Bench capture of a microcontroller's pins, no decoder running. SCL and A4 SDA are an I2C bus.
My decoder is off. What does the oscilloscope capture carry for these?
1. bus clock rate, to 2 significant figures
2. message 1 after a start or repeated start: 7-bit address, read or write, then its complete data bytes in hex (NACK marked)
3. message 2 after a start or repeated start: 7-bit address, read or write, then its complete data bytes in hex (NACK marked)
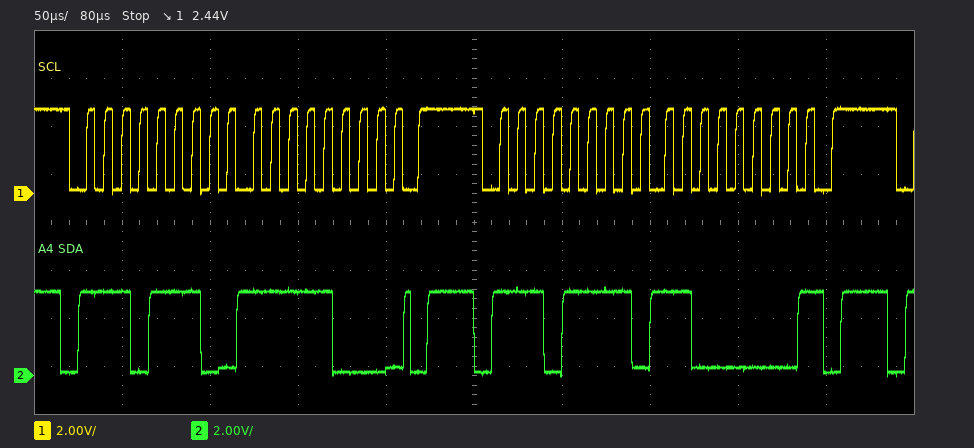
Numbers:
100 kHz
0x77 write: F8
0x77 read: C0 NACK
